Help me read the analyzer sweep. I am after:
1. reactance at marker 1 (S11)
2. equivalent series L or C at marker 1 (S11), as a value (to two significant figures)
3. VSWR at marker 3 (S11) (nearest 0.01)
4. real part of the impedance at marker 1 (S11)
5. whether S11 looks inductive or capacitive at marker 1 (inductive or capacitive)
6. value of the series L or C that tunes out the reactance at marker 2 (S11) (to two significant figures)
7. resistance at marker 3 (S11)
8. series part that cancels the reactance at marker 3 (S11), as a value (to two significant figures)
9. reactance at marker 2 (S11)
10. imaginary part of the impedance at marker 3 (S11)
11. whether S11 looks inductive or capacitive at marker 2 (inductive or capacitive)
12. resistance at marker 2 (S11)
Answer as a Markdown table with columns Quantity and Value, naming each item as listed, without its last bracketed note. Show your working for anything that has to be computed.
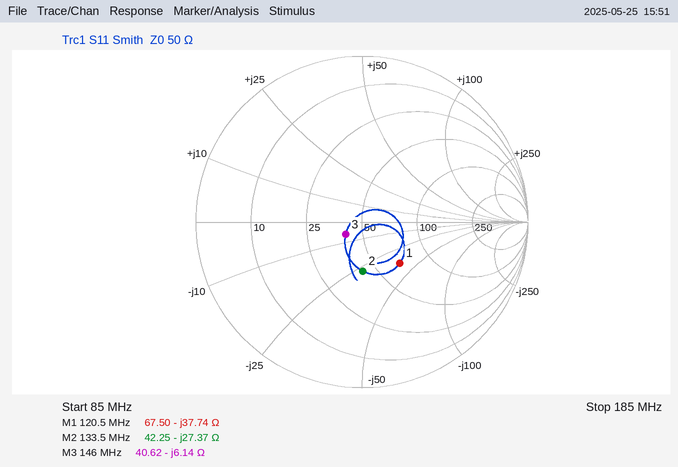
| Quantity | Value |
|---|---|
| reactance at marker 1 | -37.74 Ω |
| equivalent series L or C at marker 1 (S11), as a value | C = 1/(2π × 120.5 MHz × 37.74 Ω) ≈ 35 pF |
| VSWR at marker 3 (S11) | 1.28 |
| real part of the impedance at marker 1 | 67.50 Ω |
| whether S11 looks inductive or capacitive at marker 1 | capacitive |
| value of the series L or C that tunes out the reactance at marker 2 (S11) | L = 27.37 Ω/(2π × 133.5 MHz) ≈ 33 nH |
| resistance at marker 3 | 40.62 Ω |
| series part that cancels the reactance at marker 3 (S11), as a value | L = 6.14 Ω/(2π × 146 MHz) ≈ 6.7 nH |
| reactance at marker 2 | -27.37 Ω |
| imaginary part of the impedance at marker 3 | -6.14 Ω |
| whether S11 looks inductive or capacitive at marker 2 | capacitive |
| resistance at marker 2 | 42.25 Ω |
